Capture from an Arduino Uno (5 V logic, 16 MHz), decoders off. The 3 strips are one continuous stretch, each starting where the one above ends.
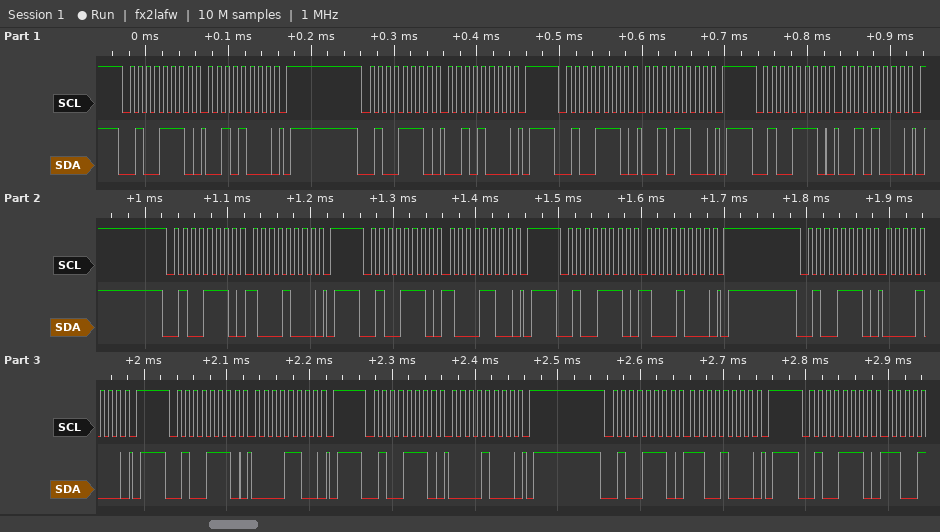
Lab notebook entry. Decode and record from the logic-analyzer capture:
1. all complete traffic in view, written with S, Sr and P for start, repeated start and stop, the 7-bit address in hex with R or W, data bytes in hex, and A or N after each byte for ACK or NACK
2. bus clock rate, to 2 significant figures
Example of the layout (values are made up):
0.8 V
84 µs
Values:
S 27W A 28 A P S 27W A 28 A P S 27W A 2C A P S 27W A 28 A P S 27W A 88 A P S 27W A 8C A P S 27W A 88 A P S 27W A 08 A P S 27W A 0C A P S 27W A 08 A P S 27W A C8 A P S 27W A
100 kHz
